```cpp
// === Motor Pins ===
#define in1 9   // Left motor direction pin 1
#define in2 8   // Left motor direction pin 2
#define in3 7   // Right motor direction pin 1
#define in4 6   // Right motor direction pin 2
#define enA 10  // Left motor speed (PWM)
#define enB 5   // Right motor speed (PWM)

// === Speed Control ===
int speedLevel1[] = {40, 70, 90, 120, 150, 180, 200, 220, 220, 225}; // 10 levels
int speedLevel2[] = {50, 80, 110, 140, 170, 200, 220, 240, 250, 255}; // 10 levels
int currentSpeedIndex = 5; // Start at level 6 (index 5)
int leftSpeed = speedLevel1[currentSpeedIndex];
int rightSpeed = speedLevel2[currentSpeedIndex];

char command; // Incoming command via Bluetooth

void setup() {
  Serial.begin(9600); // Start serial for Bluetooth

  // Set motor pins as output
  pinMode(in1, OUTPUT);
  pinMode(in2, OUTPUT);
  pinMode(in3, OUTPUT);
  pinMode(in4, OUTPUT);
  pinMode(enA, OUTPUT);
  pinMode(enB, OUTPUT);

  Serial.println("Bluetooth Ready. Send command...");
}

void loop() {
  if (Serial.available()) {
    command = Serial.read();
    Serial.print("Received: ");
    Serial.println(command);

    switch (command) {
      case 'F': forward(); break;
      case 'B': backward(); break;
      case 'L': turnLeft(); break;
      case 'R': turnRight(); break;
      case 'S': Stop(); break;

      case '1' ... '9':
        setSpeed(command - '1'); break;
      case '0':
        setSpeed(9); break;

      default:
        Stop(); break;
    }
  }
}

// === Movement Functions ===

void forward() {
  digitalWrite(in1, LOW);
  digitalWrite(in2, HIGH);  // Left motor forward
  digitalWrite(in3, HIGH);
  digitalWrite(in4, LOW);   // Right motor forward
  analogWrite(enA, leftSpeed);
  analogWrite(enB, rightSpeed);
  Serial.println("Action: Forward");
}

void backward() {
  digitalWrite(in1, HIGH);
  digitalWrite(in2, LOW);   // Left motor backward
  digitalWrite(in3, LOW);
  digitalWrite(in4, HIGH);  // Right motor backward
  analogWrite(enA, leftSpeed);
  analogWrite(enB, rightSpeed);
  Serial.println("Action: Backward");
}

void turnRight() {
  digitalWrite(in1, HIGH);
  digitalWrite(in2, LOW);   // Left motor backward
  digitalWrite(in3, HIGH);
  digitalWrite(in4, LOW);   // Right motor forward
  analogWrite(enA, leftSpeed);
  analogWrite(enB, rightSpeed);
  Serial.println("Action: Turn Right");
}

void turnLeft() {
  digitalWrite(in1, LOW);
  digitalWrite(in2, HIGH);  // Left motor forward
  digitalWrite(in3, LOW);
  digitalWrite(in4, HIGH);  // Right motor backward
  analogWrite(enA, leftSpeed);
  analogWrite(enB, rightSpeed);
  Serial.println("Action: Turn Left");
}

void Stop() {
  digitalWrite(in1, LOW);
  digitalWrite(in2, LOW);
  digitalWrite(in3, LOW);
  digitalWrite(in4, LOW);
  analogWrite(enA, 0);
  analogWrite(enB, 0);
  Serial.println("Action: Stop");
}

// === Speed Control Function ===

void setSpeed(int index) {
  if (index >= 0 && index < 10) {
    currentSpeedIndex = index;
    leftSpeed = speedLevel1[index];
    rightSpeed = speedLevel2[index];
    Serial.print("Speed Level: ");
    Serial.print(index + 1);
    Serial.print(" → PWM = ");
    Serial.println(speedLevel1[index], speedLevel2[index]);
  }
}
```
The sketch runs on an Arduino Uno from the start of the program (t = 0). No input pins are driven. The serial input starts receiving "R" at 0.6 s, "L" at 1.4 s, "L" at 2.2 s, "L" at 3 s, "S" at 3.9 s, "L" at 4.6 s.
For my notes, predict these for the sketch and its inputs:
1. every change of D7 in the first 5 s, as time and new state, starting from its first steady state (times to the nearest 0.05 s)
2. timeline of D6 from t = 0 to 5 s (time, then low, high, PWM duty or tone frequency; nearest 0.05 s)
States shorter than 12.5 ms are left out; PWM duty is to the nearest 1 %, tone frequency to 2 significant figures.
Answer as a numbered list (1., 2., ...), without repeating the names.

1. 0 s low; 0.6 s high; 1.4 s low
2. 0 s low; 1.4 s high; 3.9 s low; 4.6 s high
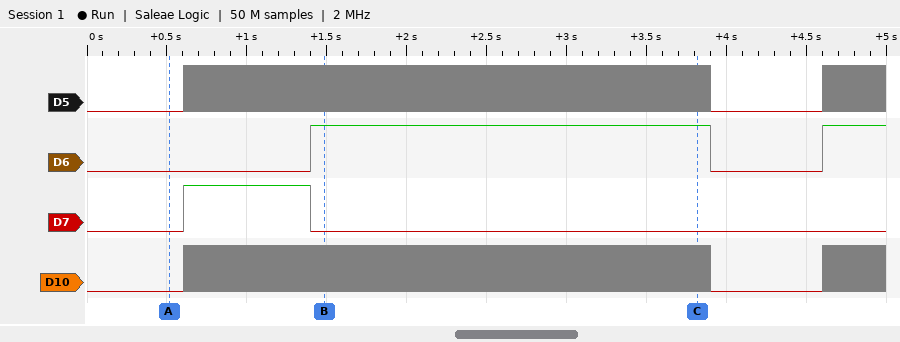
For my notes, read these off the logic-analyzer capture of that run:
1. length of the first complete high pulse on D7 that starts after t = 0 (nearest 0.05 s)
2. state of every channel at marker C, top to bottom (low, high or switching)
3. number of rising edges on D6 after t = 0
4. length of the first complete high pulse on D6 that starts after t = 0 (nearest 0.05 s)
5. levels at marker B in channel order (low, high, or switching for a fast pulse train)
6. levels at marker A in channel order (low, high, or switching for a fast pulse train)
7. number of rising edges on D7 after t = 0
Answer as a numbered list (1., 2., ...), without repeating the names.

1. 0.80 s
2. D5 switching, D6 high, D7 low, D10 switching
3. 2
4. 2.50 s
5. D5 switching, D6 high, D7 low, D10 switching
6. D5 low, D6 low, D7 low, D10 low
7. 1
